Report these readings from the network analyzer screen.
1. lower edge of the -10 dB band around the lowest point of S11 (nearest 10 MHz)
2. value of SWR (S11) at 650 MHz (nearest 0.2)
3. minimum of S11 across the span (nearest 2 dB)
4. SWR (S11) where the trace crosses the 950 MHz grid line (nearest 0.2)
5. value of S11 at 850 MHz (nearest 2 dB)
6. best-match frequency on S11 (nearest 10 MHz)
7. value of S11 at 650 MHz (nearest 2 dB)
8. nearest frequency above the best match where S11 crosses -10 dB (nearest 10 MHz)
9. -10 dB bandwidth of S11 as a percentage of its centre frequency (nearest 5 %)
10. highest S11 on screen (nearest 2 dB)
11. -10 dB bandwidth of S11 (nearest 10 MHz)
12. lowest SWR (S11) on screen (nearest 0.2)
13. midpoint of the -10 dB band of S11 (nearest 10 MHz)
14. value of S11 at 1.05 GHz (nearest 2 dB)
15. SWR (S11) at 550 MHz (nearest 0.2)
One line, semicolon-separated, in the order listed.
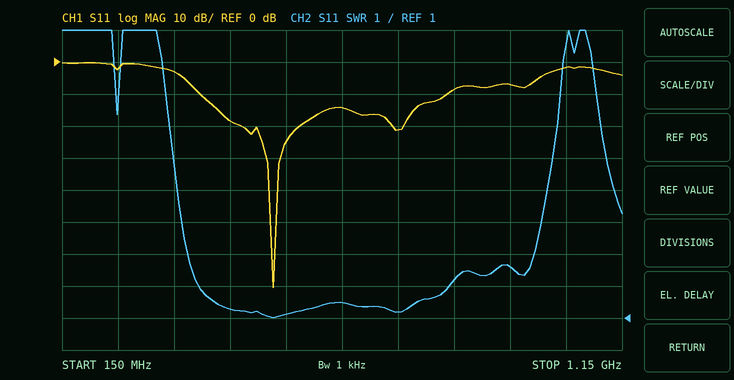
400 MHz; 1.4; -70 dB; 2.6; -8 dB; 530 MHz; -14 dB; 840 MHz; 70 %; 0 dB; 440 MHz; 1.0; 620 MHz; -2 dB; 1.2
